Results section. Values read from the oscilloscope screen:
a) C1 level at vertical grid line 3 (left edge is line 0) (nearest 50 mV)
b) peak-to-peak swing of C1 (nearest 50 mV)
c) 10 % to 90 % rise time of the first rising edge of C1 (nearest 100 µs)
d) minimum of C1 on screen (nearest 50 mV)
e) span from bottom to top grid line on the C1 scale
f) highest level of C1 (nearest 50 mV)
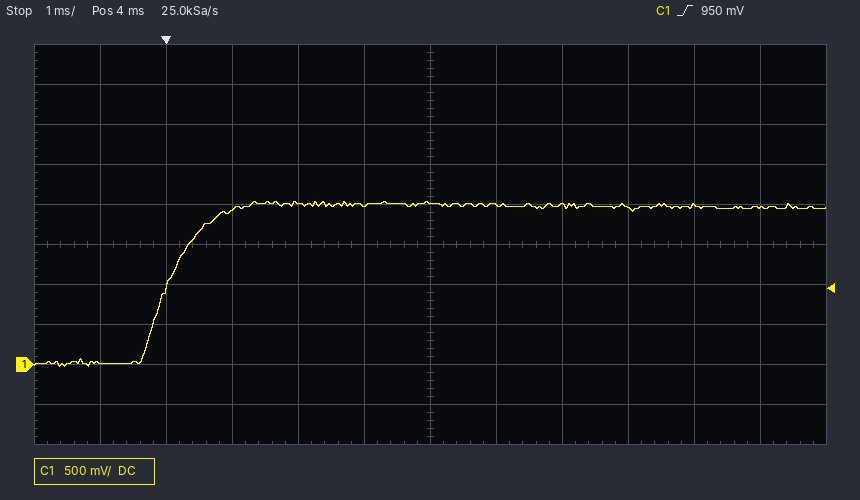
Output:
1.95 V
2.05 V
1.0 ms
0 mV
5 V
2.05 V
